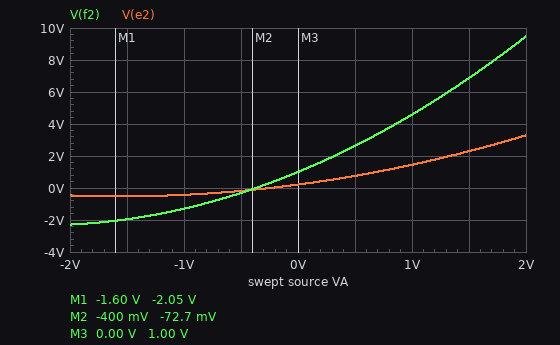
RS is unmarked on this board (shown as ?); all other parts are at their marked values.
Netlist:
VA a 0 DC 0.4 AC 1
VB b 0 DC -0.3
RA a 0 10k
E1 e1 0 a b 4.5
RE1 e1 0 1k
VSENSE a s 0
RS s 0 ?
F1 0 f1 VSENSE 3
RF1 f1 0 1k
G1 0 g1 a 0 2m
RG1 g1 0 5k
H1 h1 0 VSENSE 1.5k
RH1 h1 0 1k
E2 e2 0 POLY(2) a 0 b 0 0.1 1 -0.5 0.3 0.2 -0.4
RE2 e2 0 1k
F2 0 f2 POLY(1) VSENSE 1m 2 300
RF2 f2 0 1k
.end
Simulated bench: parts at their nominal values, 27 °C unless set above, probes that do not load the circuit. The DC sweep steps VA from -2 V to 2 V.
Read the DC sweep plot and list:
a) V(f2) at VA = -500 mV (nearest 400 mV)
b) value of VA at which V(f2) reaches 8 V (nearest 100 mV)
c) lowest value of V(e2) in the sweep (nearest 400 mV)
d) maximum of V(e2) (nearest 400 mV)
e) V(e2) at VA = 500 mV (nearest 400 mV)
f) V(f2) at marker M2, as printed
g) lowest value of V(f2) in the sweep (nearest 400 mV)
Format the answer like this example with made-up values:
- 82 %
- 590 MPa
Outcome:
- -400 mV
- 1.7 V
- -400 mV
- 3.2 V
- 800 mV
- -72.7 mV
- -2.4 V
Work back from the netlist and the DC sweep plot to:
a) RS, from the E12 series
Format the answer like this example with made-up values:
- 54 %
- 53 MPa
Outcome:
- 680 Ω
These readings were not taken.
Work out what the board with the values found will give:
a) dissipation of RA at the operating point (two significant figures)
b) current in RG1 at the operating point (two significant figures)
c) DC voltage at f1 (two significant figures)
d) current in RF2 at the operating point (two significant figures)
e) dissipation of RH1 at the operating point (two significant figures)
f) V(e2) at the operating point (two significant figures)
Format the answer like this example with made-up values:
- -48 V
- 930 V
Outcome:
- 16 µW
- 800 µA
- 1.8 V
- 2.3 mA
- 780 µW
- 640 mV
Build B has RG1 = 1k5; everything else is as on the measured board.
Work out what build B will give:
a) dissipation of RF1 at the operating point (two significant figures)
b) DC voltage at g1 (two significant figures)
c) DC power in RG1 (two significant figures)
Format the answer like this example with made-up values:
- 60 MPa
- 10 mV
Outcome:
- 3.1 mW
- 1.2 V
- 960 µW
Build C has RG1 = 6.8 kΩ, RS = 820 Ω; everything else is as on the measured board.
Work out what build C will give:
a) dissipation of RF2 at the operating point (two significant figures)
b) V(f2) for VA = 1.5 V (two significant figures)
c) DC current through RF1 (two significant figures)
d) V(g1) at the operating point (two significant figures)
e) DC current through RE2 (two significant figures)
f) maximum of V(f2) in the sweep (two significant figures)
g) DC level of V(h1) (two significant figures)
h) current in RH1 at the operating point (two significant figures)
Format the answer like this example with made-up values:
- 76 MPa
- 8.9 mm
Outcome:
- 4.2 mW
- 5.7 V
- 1.5 mA
- 5.4 V
- 640 µA
- 7.7 V
- 730 mV
- 730 µA
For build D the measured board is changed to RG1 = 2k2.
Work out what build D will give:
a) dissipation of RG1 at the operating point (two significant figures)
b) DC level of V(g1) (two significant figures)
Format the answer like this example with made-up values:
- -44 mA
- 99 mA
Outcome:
- 1.4 mW
- 1.8 V
